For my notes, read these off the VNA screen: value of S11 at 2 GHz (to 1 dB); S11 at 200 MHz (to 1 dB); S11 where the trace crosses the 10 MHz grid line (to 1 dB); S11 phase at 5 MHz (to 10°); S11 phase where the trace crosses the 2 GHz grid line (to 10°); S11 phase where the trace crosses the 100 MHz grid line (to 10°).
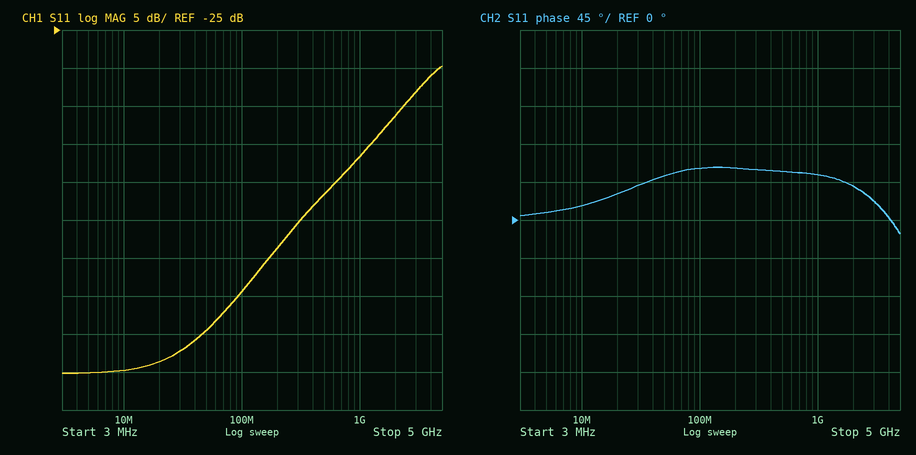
-36 dB
-54 dB
-70 dB
10°
40°
60°
